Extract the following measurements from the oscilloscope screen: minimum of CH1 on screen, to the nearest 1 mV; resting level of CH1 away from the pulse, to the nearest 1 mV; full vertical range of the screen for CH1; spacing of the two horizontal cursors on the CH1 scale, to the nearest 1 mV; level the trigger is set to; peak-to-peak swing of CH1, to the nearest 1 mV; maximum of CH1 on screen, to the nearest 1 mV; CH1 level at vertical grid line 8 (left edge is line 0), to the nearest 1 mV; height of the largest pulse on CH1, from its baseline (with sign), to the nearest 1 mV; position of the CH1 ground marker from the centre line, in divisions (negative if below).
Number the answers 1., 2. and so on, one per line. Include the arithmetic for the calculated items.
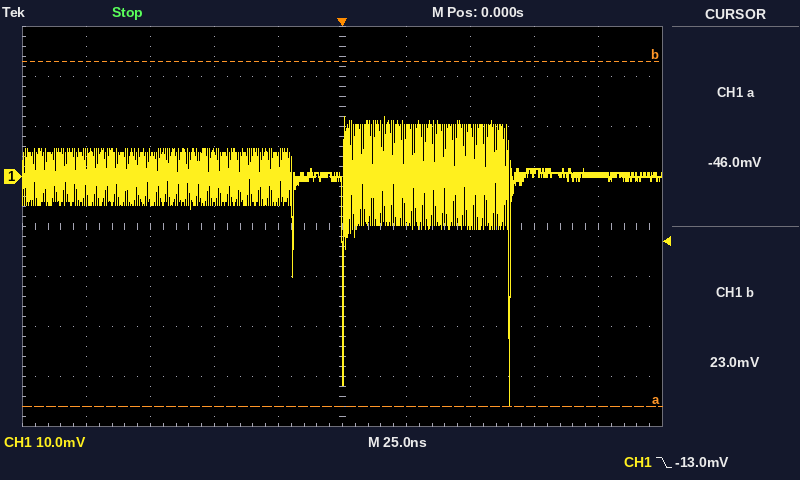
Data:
1. -46 mV
2. 0 mV
3. 80 mV
4. 69 mV
5. -13.0 mV
6. 12 mV − (-46 mV) = 58 mV
7. 12 mV
8. 1 mV
9. -46 mV − (0 mV) = -46 mV
10. +1.0 div
